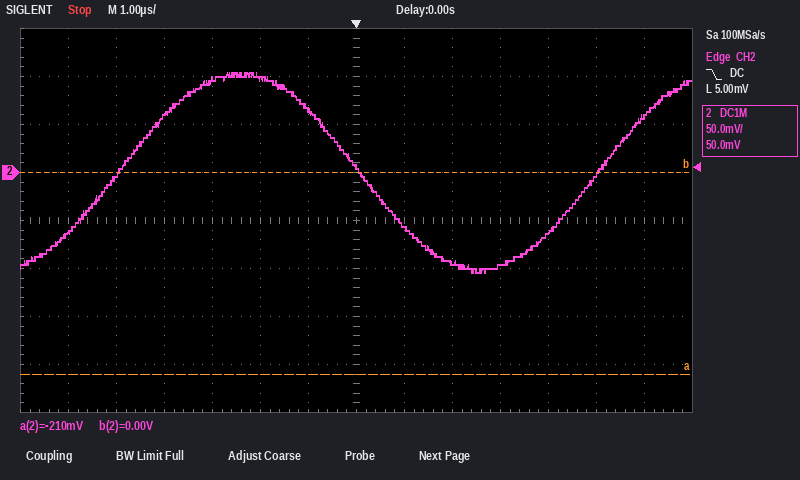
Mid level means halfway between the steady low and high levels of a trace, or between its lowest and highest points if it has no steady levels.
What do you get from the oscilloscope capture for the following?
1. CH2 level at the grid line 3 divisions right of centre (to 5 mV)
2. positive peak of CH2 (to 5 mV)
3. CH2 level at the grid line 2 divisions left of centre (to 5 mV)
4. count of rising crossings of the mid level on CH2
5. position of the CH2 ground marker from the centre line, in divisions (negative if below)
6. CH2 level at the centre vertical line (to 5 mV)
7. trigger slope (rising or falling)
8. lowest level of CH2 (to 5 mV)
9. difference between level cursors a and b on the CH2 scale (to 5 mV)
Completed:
-95 mV
105 mV
100 mV
2
+1.0 div
5 mV
falling
-105 mV
210 mV
